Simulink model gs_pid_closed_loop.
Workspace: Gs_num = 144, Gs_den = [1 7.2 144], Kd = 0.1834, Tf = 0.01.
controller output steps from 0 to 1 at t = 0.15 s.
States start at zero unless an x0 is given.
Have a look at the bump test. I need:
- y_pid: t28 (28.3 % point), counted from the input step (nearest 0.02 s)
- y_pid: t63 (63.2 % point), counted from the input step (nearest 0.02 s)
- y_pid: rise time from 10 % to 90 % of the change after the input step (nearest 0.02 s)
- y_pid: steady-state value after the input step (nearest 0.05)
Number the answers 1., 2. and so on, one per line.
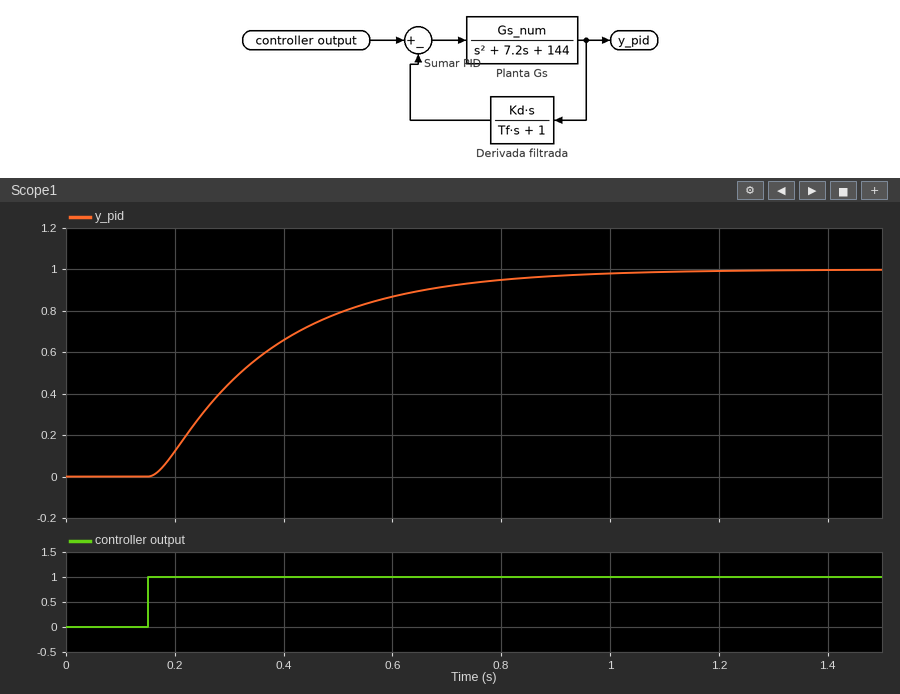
1. 0.10 s
2. 0.24 s
3. 0.46 s
4. 1.00
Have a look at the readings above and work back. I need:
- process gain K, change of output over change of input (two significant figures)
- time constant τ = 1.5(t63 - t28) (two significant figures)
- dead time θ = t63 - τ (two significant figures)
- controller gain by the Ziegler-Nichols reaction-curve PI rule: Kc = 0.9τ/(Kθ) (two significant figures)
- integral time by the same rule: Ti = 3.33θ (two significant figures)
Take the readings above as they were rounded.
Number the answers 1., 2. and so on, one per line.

1. 1.0
2. 0.21 s
3. 0.030 s
4. 6.3
5. 0.100 s
